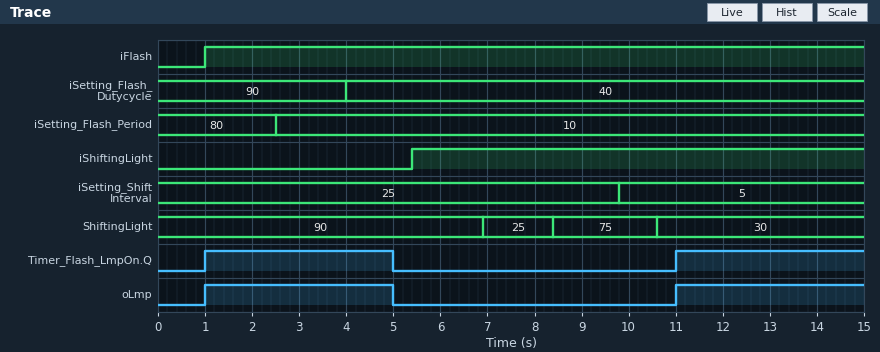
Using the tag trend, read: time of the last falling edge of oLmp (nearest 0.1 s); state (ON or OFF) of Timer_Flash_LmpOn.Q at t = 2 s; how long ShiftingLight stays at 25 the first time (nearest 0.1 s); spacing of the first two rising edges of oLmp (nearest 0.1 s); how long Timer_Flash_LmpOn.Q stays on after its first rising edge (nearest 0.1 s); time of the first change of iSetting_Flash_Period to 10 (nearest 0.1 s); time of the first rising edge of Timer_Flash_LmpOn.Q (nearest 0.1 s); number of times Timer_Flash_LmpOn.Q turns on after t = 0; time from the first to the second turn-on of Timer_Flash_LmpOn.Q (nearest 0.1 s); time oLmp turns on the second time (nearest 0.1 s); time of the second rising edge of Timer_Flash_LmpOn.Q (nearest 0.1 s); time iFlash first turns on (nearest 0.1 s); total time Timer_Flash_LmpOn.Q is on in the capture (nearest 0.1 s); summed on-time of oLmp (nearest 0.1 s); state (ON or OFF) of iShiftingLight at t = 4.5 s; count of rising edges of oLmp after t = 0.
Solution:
5.0 s
ON
1.5 s
10.0 s
4.0 s
2.5 s
1.0 s
2
10.0 s
11.0 s
11.0 s
1.0 s
8.0 s
8.0 s
OFF
2
